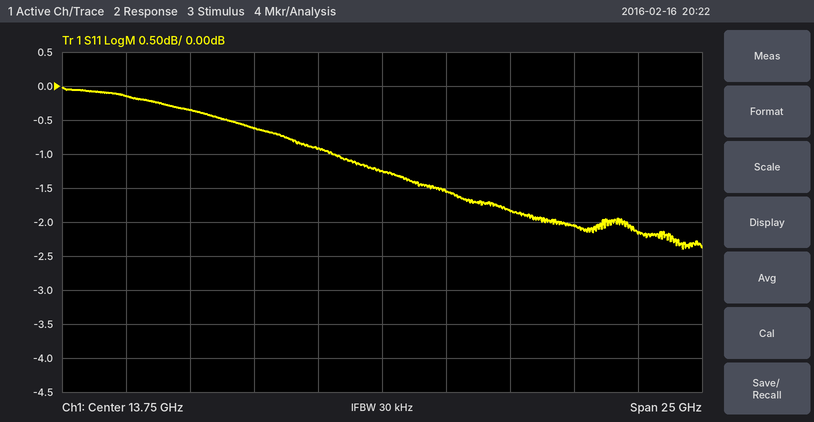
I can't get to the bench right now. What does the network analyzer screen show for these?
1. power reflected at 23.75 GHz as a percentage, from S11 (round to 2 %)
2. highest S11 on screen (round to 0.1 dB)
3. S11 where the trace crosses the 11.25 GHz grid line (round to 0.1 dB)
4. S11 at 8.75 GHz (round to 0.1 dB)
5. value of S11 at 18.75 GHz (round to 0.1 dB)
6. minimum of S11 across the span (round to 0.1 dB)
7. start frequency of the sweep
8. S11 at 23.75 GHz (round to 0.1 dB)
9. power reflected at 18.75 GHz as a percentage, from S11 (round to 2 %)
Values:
60 %
0.0 dB
-0.9 dB
-0.6 dB
-1.8 dB
-2.4 dB
1.25 GHz
-2.2 dB
66 %
